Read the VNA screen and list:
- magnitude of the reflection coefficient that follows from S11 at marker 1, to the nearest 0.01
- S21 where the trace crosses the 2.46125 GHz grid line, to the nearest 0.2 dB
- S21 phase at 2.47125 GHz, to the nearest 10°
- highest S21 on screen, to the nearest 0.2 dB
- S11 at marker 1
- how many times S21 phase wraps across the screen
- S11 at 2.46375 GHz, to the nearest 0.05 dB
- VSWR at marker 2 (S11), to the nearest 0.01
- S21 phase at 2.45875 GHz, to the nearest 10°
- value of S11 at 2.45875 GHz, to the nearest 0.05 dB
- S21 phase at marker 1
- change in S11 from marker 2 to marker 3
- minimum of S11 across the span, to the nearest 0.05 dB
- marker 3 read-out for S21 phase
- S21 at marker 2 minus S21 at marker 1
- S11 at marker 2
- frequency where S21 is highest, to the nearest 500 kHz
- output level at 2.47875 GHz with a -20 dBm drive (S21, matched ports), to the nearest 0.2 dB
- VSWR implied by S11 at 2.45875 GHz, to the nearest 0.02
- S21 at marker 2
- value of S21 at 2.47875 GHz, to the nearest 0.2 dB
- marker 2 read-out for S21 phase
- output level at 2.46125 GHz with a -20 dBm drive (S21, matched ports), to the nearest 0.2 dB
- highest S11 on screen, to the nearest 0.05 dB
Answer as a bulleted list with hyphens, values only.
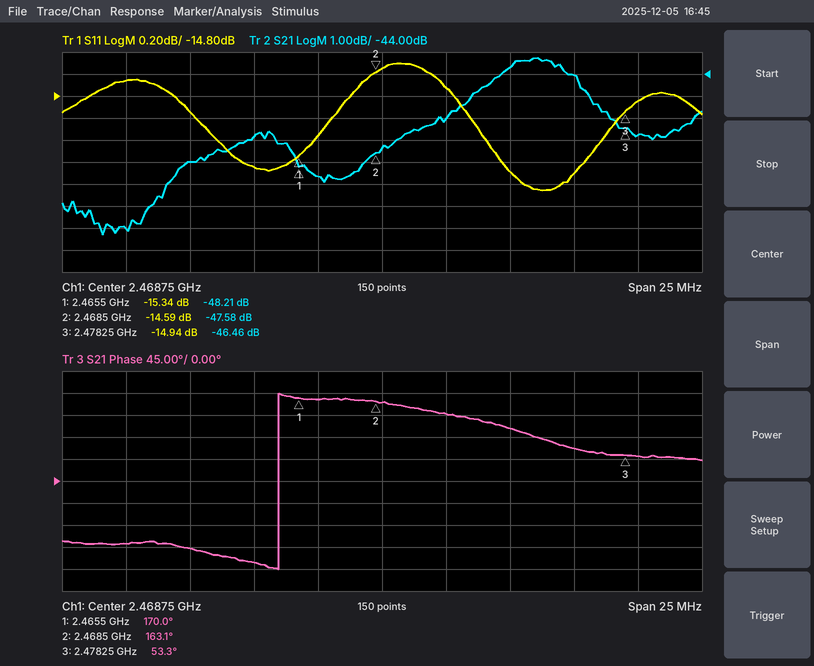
- 0.17
- -48.0 dB
- 140°
- -43.2 dB
- -15.34 dB
- 1
- -15.45 dB
- 1.46
- -130°
- -14.65 dB
- 170.0°
- -0.35 dB
- -15.65 dB
- 53.3°
- 0.63 dB
- -14.59 dB
- 2.4750 GHz
- -66.8 dBm
- 1.46
- -47.58 dB
- -46.8 dB
- 163.1°
- -68.0 dBm
- -14.50 dB
